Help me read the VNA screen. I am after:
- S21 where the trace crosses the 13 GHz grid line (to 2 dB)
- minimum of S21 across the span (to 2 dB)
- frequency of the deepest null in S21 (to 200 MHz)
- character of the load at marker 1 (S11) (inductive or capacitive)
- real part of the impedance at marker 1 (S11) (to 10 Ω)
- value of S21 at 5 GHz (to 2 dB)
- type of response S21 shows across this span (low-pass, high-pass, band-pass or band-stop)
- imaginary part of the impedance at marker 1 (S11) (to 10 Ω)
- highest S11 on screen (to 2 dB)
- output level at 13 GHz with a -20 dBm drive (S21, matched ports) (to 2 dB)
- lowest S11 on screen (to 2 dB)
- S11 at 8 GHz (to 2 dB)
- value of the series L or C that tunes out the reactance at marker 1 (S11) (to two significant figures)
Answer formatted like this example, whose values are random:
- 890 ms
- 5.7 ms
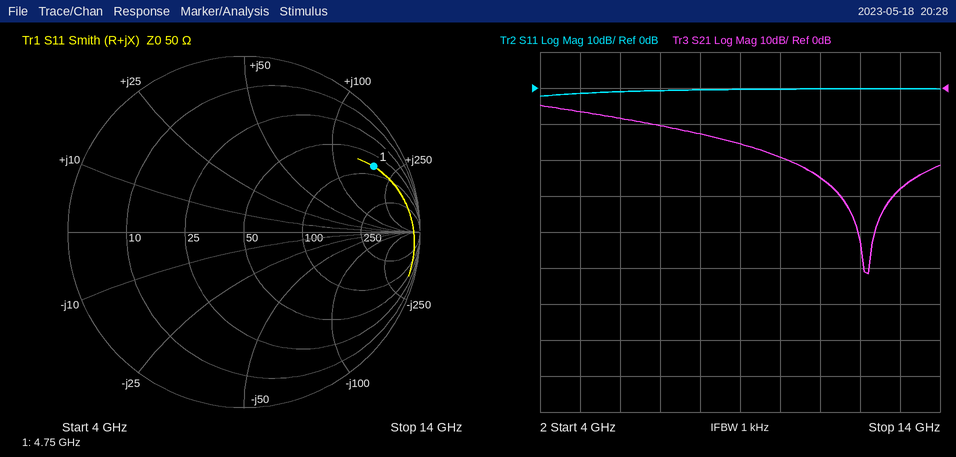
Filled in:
- -28 dB
- -52 dB
- 12.2 GHz
- inductive
- 80 Ω
- -6 dB
- low-pass
- +180 Ω
- 0 dB
- -48 dBm
- -2 dB
- 0 dB
- 190 fF
